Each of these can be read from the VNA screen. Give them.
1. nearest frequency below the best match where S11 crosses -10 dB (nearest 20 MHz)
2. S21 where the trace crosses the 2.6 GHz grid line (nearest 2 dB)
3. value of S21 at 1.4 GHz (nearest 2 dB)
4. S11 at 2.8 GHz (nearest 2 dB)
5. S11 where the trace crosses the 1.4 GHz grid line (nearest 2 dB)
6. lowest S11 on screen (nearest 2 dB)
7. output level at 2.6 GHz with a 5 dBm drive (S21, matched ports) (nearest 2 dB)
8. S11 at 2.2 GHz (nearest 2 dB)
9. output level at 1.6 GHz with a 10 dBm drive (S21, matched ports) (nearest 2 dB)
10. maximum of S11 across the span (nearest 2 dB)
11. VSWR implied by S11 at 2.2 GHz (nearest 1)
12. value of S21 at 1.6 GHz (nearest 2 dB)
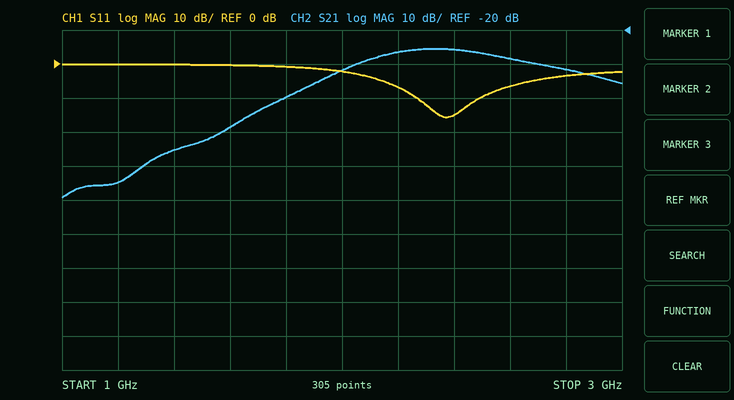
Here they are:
2.26 GHz
-28 dB
-56 dB
-4 dB
0 dB
-16 dB
-24 dBm
-6 dB
-38 dBm
0 dB
3
-48 dB
